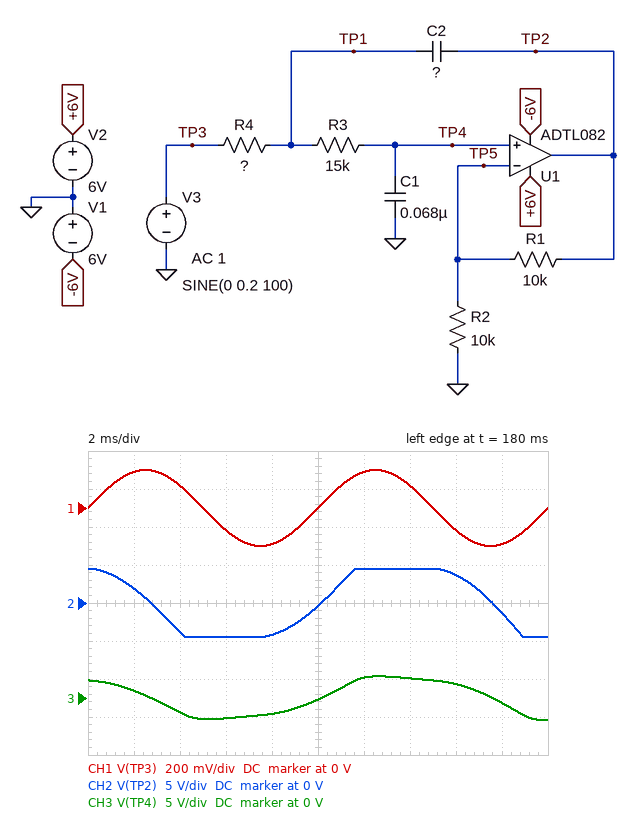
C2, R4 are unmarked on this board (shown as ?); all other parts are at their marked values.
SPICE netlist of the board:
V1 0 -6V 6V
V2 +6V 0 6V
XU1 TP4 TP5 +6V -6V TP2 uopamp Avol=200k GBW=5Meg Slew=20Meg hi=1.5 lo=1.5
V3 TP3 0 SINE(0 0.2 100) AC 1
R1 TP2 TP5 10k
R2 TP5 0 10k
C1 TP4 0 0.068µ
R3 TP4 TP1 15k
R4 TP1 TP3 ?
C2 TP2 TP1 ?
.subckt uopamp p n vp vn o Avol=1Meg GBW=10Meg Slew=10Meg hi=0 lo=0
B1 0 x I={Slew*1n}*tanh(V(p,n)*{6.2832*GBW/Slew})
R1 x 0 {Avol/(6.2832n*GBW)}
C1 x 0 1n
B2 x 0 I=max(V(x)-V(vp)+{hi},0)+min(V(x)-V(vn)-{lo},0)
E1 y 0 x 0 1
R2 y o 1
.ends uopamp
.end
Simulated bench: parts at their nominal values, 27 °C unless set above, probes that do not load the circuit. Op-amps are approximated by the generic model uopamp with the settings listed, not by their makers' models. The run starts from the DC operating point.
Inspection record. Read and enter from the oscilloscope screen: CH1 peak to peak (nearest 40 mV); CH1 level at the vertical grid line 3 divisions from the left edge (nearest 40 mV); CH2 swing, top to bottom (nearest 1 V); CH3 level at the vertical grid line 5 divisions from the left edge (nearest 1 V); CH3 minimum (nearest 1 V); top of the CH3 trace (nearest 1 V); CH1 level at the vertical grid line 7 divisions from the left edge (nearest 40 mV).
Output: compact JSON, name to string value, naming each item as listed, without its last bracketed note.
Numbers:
{"CH1 peak to peak": "400 mV", "CH1 level at the vertical grid line 3 divisions from the left edge": "-120 mV", "CH2 swing, top to bottom": "9 V", "CH3 level at the vertical grid line 5 divisions from the left edge": "0 V", "CH3 minimum": "-3 V", "top of the CH3 trace": "3 V", "CH1 level at the vertical grid line 7 divisions from the left edge": "120 mV"}
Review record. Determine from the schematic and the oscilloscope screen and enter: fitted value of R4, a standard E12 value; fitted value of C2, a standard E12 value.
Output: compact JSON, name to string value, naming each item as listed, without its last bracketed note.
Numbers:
{"fitted value of R4, a standard E12 value": "39 kΩ", "fitted value of C2, a standard E12 value": "120 nF"}
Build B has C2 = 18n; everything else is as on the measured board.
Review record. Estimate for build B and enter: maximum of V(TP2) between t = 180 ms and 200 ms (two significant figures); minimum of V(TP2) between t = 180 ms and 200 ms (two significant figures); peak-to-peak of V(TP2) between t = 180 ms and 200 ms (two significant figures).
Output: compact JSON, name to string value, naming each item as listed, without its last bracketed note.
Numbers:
{"maximum of V(TP2) between t = 180 ms and 200 ms": "200 mV", "minimum of V(TP2) between t = 180 ms and 200 ms": "-200 mV", "peak-to-peak of V(TP2) between t = 180 ms and 200 ms": "400 mV"}
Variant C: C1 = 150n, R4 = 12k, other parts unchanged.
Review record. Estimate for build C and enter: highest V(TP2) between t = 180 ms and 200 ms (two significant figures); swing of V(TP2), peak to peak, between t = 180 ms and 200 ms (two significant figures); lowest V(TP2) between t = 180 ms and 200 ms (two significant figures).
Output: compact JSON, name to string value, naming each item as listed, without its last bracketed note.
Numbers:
{"highest V(TP2) between t = 180 ms and 200 ms": "240 mV", "swing of V(TP2), peak to peak, between t = 180 ms and 200 ms": "480 mV", "lowest V(TP2) between t = 180 ms and 200 ms": "-240 mV"}
